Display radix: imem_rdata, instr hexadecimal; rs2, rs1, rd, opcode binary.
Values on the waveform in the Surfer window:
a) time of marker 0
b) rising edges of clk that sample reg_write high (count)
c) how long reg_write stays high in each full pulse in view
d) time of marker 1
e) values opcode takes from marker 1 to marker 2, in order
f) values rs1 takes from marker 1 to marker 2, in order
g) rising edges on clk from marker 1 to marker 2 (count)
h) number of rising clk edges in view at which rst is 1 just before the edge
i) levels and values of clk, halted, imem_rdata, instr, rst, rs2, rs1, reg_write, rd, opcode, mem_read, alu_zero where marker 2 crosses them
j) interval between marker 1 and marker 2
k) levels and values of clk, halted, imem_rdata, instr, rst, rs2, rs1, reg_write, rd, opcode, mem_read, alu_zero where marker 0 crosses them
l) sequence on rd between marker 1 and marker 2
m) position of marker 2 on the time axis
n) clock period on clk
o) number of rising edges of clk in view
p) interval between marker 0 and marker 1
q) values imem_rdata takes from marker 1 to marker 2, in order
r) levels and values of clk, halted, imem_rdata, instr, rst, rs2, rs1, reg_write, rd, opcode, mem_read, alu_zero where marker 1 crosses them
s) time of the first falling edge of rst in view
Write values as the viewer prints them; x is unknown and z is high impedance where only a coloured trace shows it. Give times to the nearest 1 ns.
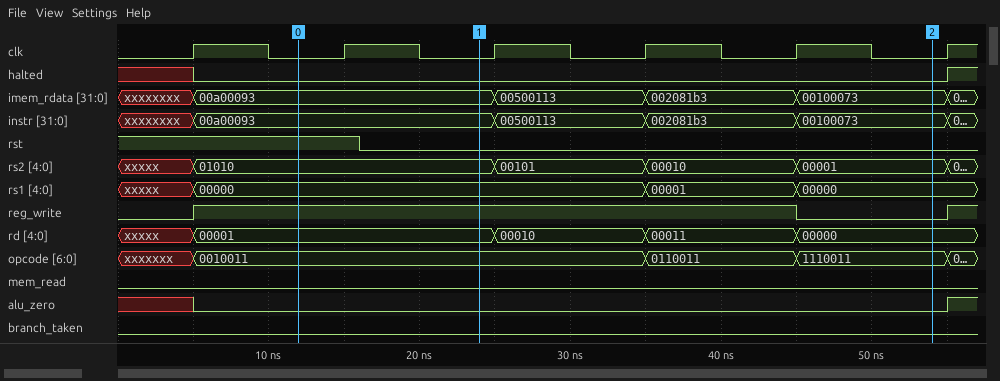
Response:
12 ns
4
40 ns
24 ns
0010011, 0110011, 1110011
00000, 00001, 00000
3
2
clk=0, halted=0, imem_rdata=00100073, instr=00100073, rst=0, rs2=00001, rs1=00000, reg_write=0, rd=00000, opcode=1110011, mem_read=0, alu_zero=0
30 ns
clk=0, halted=0, imem_rdata=00a00093, instr=00a00093, rst=1, rs2=01010, rs1=00000, reg_write=1, rd=00001, opcode=0010011, mem_read=0, alu_zero=0
00001, 00010, 00011, 00000
54 ns
10 ns
6
12 ns
00a00093, 00500113, 002081b3, 00100073
clk=0, halted=0, imem_rdata=00a00093, instr=00a00093, rst=0, rs2=01010, rs1=00000, reg_write=1, rd=00001, opcode=0010011, mem_read=0, alu_zero=0
16 ns
